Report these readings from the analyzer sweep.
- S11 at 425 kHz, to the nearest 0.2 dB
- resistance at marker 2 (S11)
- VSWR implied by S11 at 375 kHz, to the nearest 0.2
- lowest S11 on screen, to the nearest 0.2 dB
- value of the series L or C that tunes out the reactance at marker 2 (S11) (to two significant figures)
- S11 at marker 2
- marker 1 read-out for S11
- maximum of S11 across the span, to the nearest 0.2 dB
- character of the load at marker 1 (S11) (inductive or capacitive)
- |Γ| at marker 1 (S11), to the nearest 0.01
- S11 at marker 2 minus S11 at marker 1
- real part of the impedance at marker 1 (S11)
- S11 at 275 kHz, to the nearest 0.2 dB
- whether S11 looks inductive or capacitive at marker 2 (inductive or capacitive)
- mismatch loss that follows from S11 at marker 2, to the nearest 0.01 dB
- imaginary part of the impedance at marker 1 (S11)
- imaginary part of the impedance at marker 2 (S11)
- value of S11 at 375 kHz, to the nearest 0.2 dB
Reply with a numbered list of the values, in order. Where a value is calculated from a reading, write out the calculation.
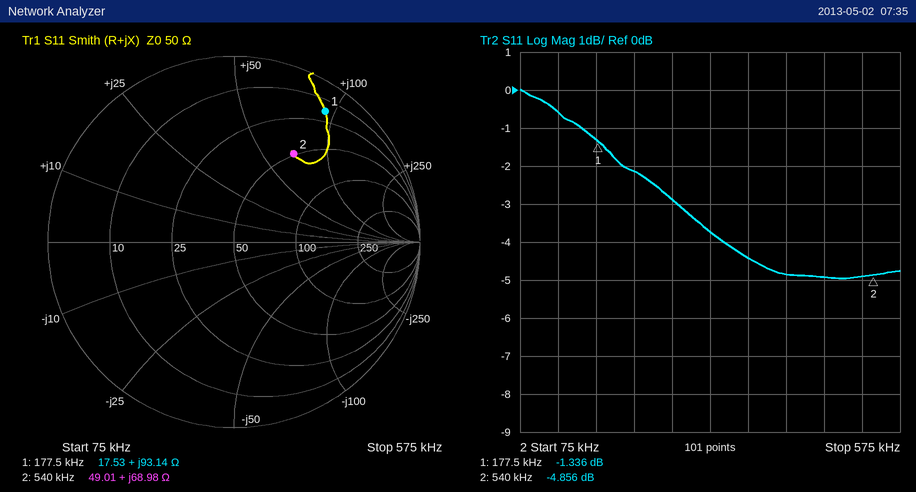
1. -4.8 dB
2. 49.01 Ω
3. |Γ| = 10^(-4.4/20) = 0.6026; VSWR = (1 + 0.6026)/(1 − 0.6026) ≈ 4.0
4. -5.0 dB
5. C = 1/(2π × 540 kHz × 68.98 Ω) ≈ 4.3 nF
6. -4.856 dB
7. -1.336 dB
8. 0.0 dB
9. inductive
10. 0.86
11. -4.856 − (-1.336) = -3.520 dB
12. 17.53 Ω
13. -2.8 dB
14. inductive
15. −10 log10(1 − 10^(-4.856/10)) ≈ 1.72 dB
16. +93.14 Ω
17. +68.98 Ω
18. -4.4 dB
